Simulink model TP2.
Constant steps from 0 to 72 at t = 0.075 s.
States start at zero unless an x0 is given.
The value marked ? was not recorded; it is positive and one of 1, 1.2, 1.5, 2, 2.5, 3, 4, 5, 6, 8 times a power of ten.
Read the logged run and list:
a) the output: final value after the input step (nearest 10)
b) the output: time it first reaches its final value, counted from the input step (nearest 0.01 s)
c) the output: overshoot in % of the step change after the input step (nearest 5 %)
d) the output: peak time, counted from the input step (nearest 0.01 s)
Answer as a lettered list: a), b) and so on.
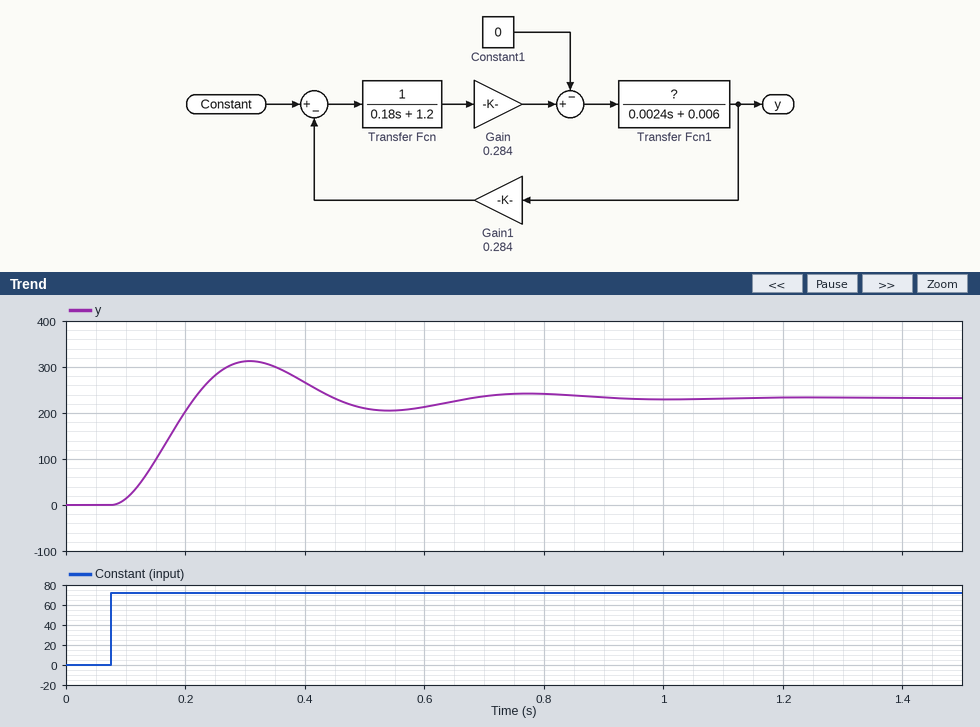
a) 230
b) 0.14 s
c) 35 %
d) 0.23 s
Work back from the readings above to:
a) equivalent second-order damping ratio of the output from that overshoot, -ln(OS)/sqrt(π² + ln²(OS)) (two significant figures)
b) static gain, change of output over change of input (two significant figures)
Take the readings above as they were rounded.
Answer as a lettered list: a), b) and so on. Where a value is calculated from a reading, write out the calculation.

a) ln(0.35) = -1.050; 1.050 / sqrt(9.870 + 1.102) = 0.32
b) (230 - 0) / (72 - 0) = 3.2
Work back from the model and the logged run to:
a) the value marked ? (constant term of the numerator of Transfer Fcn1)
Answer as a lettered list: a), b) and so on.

a) 1
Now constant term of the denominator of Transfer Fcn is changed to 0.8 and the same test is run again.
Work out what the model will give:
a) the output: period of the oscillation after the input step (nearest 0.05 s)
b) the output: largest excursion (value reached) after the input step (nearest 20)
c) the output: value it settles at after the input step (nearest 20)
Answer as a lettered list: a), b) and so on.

a) 0.45 s
b) 340
c) 240
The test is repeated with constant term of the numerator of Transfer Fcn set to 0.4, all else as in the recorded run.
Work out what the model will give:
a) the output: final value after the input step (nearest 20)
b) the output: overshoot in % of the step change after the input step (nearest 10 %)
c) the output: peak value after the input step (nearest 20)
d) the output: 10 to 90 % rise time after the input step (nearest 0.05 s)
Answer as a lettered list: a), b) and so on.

a) 200
b) 20 %
c) 240
d) 0.15 s
